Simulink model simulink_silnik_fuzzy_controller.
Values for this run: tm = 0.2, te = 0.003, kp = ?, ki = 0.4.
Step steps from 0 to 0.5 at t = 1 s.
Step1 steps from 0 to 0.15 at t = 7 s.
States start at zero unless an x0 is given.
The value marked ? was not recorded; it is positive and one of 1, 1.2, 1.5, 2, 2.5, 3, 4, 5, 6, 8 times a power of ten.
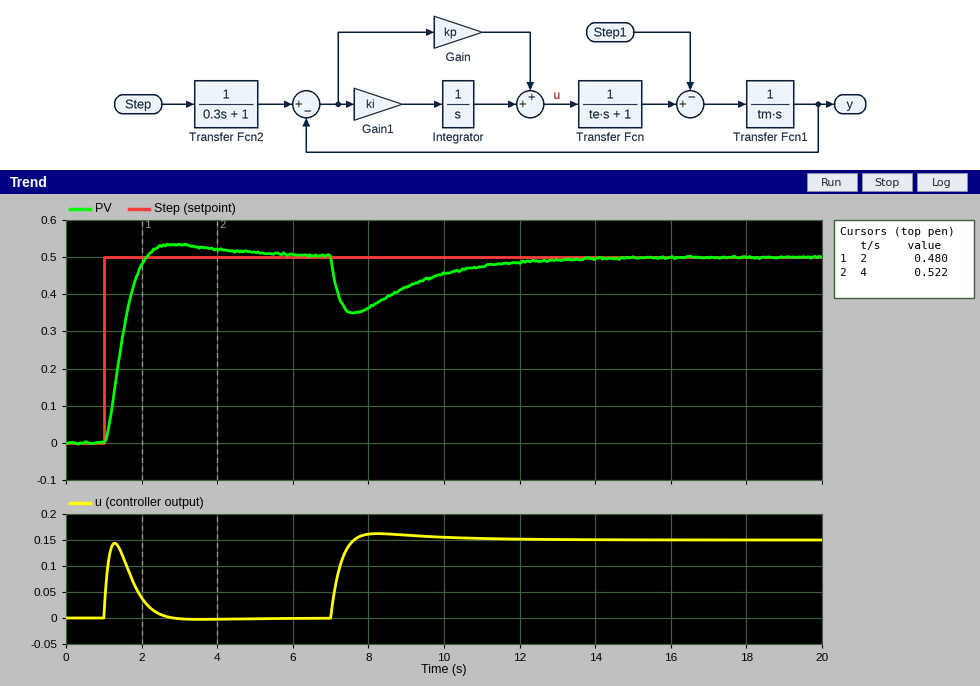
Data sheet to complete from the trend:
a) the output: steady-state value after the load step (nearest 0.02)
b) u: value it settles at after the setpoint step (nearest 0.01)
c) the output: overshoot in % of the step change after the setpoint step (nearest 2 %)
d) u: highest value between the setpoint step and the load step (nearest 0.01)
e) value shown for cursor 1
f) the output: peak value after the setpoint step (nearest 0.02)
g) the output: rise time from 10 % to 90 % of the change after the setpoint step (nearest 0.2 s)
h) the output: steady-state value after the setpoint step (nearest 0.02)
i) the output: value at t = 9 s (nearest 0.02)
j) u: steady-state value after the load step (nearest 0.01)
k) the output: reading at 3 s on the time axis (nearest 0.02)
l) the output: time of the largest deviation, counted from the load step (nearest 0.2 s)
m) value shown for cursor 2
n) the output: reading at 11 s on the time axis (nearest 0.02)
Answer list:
0.50
0.00
6 %
0.14
0.480
0.54
0.8 s
0.50
0.42
0.15
0.54
0.6 s
0.522
0.48
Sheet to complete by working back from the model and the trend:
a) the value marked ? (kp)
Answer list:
0.8
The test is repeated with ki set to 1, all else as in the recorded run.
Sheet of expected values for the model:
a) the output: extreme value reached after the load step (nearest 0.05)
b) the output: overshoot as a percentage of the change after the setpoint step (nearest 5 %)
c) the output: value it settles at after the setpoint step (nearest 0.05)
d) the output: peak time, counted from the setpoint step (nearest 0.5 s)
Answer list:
0.35
10 %
0.50
1.5 s
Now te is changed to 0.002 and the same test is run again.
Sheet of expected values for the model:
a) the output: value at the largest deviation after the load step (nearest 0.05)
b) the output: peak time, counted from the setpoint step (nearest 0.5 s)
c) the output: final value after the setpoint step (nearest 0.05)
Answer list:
0.35
2.0 s
0.50
